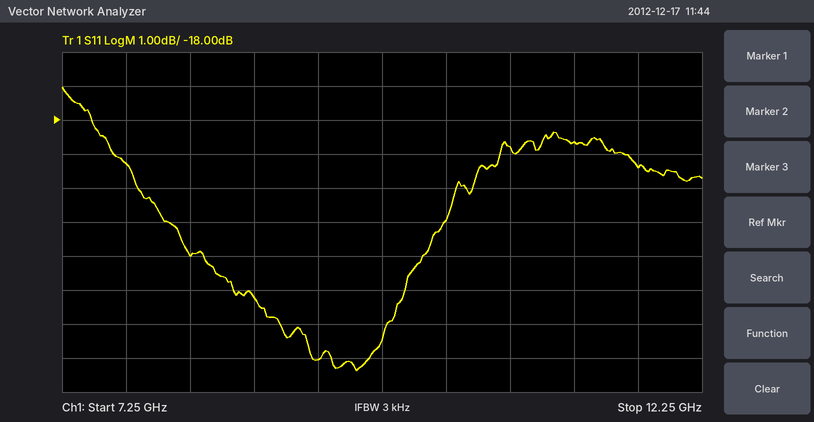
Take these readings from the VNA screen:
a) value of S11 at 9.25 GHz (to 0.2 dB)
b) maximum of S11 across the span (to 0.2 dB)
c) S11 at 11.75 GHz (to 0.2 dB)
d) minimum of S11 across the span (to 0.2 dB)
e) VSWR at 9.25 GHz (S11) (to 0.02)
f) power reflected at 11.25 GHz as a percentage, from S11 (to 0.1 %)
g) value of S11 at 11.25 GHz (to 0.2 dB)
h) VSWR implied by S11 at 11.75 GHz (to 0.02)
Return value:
-25.0 dB
-17.0 dB
-19.4 dB
-25.4 dB
1.12
1.4 %
-18.6 dB
1.24
